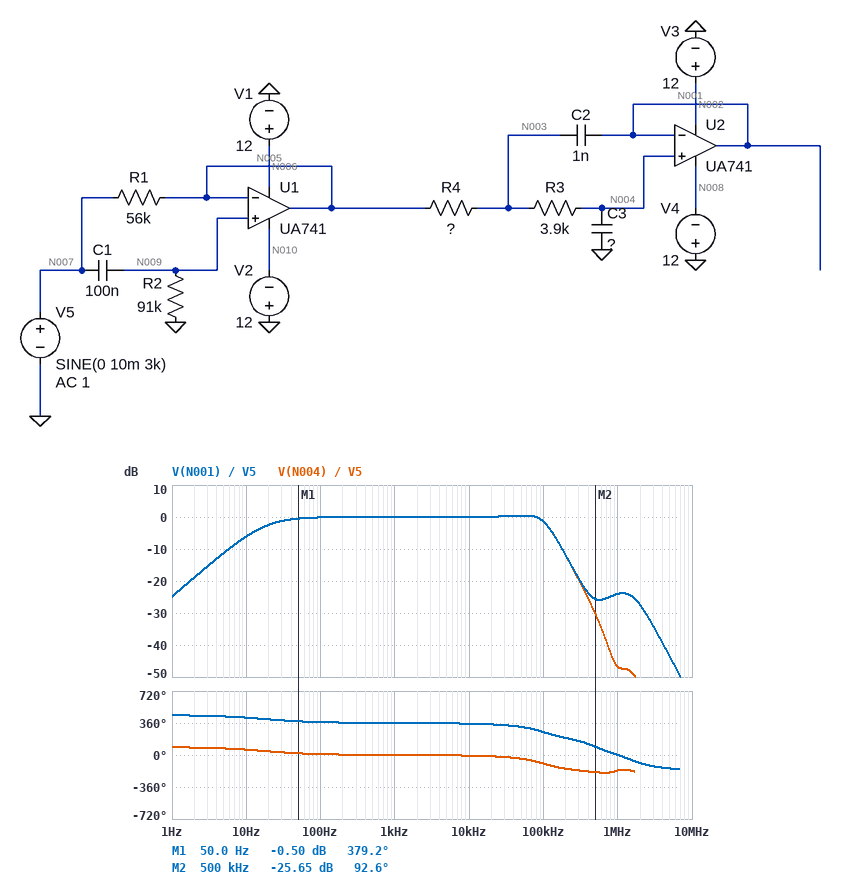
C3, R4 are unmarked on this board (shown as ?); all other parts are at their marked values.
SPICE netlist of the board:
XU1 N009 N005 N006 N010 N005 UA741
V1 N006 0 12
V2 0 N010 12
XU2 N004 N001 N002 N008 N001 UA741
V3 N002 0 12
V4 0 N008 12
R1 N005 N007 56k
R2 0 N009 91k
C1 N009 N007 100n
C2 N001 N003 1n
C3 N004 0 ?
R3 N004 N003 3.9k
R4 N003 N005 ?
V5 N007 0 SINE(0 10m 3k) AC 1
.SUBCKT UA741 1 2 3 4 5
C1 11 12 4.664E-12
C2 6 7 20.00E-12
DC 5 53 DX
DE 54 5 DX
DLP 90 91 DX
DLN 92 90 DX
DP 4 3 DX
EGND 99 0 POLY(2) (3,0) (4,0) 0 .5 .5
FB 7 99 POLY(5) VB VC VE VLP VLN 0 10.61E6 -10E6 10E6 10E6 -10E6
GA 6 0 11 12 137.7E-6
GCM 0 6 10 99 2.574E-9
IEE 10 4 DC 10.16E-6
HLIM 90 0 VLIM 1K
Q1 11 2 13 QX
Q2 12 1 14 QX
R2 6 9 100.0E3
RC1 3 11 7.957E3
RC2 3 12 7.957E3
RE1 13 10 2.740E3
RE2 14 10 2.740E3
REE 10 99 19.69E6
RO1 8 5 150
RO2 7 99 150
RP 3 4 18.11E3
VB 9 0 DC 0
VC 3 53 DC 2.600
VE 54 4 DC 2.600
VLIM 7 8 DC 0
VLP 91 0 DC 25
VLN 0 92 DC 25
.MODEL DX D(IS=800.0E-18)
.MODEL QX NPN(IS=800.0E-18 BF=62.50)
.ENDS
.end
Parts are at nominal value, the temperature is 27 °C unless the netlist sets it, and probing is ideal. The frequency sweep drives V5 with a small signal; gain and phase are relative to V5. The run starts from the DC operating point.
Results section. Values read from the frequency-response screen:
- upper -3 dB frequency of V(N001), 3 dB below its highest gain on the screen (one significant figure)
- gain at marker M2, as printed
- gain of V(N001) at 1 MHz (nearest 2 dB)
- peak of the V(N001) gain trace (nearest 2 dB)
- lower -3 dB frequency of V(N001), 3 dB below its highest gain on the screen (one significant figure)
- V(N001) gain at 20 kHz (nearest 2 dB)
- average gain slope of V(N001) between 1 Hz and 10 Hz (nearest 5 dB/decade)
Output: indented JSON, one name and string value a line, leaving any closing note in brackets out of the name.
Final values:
{
  "upper -3 dB frequency of V(N001), 3 dB below its highest gain on the screen": "100 kHz",
  "gain at marker M2, as printed": "-25.65 dB",
  "gain of V(N001) at 1 MHz": "-24 dB",
  "peak of the V(N001) gain trace": "0 dB",
  "lower -3 dB frequency of V(N001), 3 dB below its highest gain on the screen": "20 Hz",
  "V(N001) gain at 20 kHz": "0 dB",
  "average gain slope of V(N001) between 1 Hz and 10 Hz": "20 dB/decade"
}
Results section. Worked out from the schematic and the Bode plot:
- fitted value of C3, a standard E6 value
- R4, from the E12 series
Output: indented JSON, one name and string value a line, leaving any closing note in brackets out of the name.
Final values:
{
  "fitted value of C3, a standard E6 value": "330 pF",
  "R4, from the E12 series": "1.8 kΩ"
}
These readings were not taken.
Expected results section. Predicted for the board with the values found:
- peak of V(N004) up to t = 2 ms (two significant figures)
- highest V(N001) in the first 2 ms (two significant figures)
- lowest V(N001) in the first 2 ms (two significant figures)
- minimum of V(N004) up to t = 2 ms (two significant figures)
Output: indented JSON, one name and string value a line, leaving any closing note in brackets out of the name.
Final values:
{
  "peak of V(N004) up to t = 2 ms": "2.3 mV",
  "highest V(N001) in the first 2 ms": "2.3 mV",
  "lowest V(N001) in the first 2 ms": "-18 mV",
  "minimum of V(N004) up to t = 2 ms": "-18 mV"
}
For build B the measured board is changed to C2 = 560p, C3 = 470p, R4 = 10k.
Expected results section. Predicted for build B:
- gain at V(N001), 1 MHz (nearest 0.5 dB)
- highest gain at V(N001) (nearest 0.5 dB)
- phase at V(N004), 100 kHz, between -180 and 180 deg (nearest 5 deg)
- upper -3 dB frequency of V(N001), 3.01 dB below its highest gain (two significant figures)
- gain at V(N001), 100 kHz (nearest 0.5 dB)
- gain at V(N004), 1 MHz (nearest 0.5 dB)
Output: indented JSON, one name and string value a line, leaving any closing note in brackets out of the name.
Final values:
{
  "gain at V(N001), 1 MHz": "-38.0 dB",
  "highest gain at V(N001)": "0 dB",
  "phase at V(N004), 100 kHz, between -180 and 180 deg": "-135 deg",
  "upper -3 dB frequency of V(N001), 3.01 dB below its highest gain": "32 kHz",
  "gain at V(N001), 100 kHz": "-14.5 dB",
  "gain at V(N004), 1 MHz": "-57.5 dB"
}
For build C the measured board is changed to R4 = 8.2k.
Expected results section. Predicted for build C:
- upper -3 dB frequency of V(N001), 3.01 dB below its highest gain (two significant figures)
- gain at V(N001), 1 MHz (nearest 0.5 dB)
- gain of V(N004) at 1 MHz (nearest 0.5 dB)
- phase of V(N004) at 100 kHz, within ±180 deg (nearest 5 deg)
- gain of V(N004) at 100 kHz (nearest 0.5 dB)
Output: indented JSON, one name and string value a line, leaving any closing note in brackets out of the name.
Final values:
{
  "upper -3 dB frequency of V(N001), 3.01 dB below its highest gain": "52 kHz",
  "gain at V(N001), 1 MHz": "-36.5 dB",
  "gain of V(N004) at 1 MHz": "-59.5 dB",
  "phase of V(N004) at 100 kHz, within ±180 deg": "-150 deg",
  "gain of V(N004) at 100 kHz": "-13.0 dB"
}
